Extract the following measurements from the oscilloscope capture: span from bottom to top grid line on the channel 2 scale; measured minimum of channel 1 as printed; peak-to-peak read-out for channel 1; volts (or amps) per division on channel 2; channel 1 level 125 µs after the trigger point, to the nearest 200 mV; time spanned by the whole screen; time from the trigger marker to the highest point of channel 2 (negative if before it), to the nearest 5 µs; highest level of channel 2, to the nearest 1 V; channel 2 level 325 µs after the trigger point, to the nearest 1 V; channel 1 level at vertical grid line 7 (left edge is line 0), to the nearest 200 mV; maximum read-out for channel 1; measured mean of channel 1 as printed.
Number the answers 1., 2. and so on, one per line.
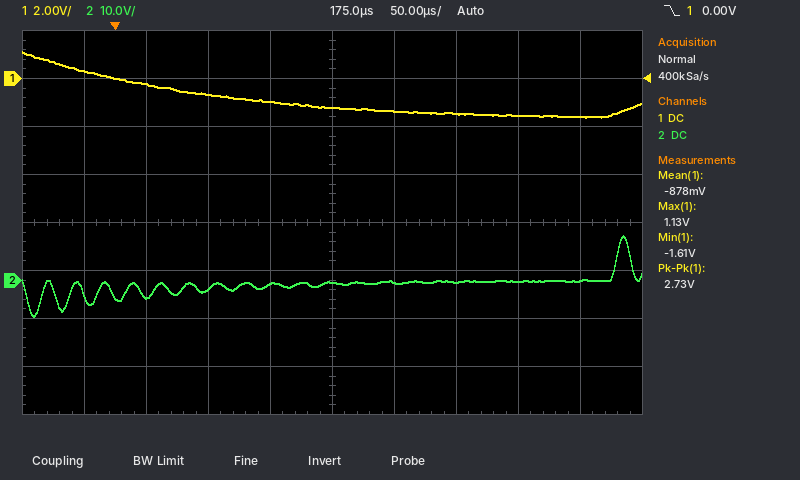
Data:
1. 80 V
2. -1.61 V
3. 2.73 V
4. 10 V
5. -1.0 V
6. 500 µs
7. +410 µs
8. 9 V
9. 0 V
10. -1.4 V
11. 1.13 V
12. -878 mV
